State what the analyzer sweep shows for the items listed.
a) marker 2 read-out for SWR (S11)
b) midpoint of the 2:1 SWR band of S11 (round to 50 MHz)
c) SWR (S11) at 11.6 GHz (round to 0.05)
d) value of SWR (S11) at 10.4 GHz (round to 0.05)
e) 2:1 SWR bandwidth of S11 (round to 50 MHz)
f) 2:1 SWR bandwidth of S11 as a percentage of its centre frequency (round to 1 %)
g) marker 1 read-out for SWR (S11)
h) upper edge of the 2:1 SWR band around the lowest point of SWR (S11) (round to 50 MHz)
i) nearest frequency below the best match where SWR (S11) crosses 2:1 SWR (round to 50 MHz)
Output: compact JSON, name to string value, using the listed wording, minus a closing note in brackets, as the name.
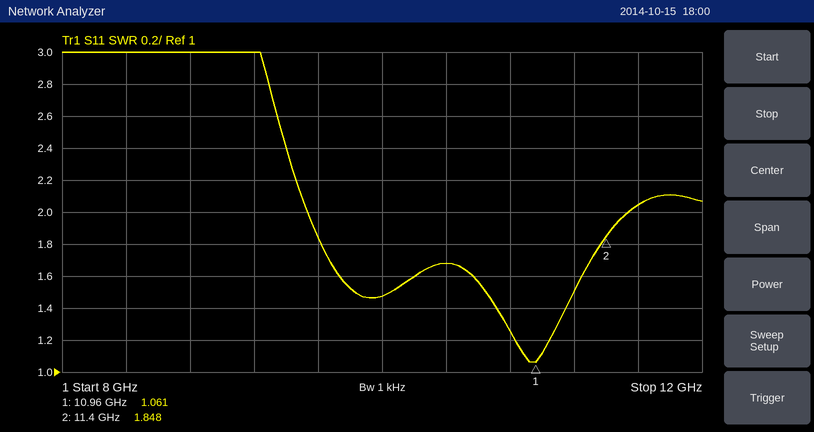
{"marker 2 read-out for SWR": "1.848", "midpoint of the 2:1 SWR band of S11": "10.55 GHz", "SWR (S11) at 11.6 GHz": "2.05", "value of SWR (S11) at 10.4 GHz": "1.70", "2:1 SWR bandwidth of S11": "2.00 GHz", "2:1 SWR bandwidth of S11 as a percentage of its centre frequency": "19 %", "marker 1 read-out for SWR": "1.061", "upper edge of the 2:1 SWR band around the lowest point of SWR (S11)": "11.55 GHz", "nearest frequency below the best match where SWR (S11) crosses 2:1 SWR": "9.55 GHz"}
